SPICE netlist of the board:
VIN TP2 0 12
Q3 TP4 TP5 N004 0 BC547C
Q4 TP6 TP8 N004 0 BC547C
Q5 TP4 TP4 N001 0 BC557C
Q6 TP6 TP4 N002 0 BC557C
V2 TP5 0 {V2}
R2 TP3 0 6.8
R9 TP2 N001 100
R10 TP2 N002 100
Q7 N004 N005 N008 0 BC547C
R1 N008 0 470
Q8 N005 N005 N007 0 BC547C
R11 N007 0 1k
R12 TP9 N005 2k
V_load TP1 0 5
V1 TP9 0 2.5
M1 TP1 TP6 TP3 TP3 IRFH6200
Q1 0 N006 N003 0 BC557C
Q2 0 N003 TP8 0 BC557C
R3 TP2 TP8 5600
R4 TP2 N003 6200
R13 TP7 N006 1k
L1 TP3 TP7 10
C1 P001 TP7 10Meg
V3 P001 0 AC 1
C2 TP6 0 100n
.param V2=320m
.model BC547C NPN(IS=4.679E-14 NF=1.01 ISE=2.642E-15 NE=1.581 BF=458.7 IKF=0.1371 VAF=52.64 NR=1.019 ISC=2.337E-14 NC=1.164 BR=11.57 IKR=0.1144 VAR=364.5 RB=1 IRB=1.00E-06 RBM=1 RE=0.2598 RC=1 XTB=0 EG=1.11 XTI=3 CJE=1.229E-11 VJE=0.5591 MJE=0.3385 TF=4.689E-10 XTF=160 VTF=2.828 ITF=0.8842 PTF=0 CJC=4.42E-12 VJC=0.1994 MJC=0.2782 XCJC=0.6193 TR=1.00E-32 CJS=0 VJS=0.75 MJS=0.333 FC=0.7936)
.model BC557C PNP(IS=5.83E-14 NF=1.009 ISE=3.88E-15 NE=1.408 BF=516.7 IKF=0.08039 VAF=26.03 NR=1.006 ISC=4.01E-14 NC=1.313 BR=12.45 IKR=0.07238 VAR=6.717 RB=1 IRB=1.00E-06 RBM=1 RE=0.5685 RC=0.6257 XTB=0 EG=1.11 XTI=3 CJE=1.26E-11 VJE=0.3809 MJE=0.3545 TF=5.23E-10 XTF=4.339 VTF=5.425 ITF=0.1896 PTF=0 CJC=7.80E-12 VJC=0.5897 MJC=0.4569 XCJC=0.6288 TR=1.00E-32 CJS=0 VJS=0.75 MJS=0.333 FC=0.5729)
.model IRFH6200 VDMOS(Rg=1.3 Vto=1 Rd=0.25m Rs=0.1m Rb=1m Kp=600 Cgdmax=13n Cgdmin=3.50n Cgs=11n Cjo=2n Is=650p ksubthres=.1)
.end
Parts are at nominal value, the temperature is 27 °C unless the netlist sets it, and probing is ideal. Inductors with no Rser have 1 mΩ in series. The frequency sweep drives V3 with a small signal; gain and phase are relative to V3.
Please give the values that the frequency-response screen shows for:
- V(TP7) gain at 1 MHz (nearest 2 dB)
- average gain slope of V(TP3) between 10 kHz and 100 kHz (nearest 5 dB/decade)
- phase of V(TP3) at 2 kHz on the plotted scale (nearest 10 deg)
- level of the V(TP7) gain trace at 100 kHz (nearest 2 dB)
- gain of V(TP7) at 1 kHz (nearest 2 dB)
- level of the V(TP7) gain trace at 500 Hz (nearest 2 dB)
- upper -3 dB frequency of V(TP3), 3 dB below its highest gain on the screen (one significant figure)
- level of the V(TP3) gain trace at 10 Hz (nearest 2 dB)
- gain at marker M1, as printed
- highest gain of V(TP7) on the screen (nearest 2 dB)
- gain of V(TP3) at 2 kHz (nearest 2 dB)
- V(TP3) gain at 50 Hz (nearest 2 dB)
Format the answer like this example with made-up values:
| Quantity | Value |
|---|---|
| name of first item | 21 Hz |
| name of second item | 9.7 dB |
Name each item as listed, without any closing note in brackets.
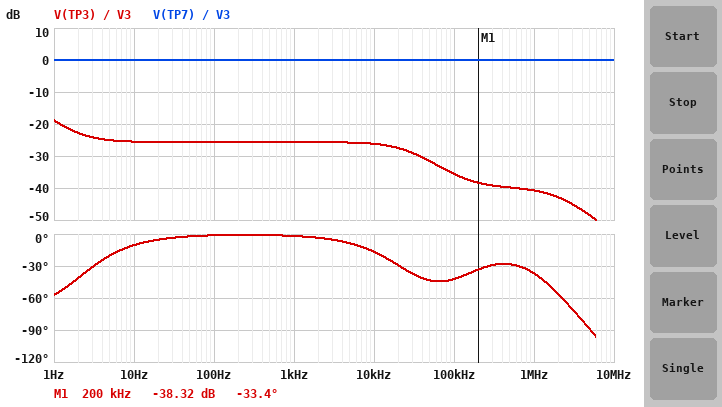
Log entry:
| Quantity | Value |
|---|---|
| V(TP7) gain at 1 MHz | 0 dB |
| average gain slope of V(TP3) between 10 kHz and 100 kHz | -10 dB/decade |
| phase of V(TP3) at 2 kHz on the plotted scale | 0 deg |
| level of the V(TP7) gain trace at 100 kHz | 0 dB |
| gain of V(TP7) at 1 kHz | 0 dB |
| level of the V(TP7) gain trace at 500 Hz | 0 dB |
| upper -3 dB frequency of V(TP3), 3 dB below its highest gain on the screen | 2 Hz |
| level of the V(TP3) gain trace at 10 Hz | -26 dB |
| gain at marker M1, as printed | -38.32 dB |
| highest gain of V(TP7) on the screen | 0 dB |
| gain of V(TP3) at 2 kHz | -26 dB |
| V(TP3) gain at 50 Hz | -26 dB |
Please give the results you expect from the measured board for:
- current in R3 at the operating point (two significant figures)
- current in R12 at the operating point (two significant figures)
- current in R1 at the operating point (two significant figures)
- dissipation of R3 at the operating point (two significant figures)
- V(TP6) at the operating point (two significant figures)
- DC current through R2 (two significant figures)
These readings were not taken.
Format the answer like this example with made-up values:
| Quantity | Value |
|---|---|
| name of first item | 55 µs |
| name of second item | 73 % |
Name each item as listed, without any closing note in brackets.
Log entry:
| Quantity | Value |
|---|---|
| current in R3 at the operating point | 1.9 mA |
| current in R12 at the operating point | 660 µA |
| current in R1 at the operating point | 1.2 mA |
| dissipation of R3 at the operating point | 21 mW |
| V(TP6) at the operating point | 570 mV |
| DC current through R2 | 480 µA |
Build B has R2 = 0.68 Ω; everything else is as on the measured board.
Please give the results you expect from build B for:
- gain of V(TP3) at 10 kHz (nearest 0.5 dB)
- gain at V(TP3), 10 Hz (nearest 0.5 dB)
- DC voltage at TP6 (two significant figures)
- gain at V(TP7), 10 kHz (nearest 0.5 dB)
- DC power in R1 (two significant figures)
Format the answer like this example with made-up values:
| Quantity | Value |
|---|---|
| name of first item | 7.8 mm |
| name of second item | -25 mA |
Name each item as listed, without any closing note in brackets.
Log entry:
| Quantity | Value |
|---|---|
| gain of V(TP3) at 10 kHz | -45.5 dB |
| gain at V(TP3), 10 Hz | -45.0 dB |
| DC voltage at TP6 | 560 mV |
| gain at V(TP7), 10 kHz | 0 dB |
| DC power in R1 | 630 µW |
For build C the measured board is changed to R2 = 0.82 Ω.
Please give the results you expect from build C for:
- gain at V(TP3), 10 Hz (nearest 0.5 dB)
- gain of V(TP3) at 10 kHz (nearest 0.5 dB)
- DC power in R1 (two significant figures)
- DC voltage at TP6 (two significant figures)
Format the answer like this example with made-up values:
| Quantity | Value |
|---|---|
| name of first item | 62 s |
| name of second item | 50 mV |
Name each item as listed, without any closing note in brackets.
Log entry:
| Quantity | Value |
|---|---|
| gain at V(TP3), 10 Hz | -43.5 dB |
| gain of V(TP3) at 10 kHz | -44.0 dB |
| DC power in R1 | 630 µW |
| DC voltage at TP6 | 560 mV |
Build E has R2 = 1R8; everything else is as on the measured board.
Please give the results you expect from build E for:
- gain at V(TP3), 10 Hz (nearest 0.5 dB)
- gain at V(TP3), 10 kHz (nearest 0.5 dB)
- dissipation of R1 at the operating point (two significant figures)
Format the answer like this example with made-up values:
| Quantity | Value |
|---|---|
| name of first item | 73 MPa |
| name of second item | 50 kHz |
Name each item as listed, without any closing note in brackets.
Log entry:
| Quantity | Value |
|---|---|
| gain at V(TP3), 10 Hz | -36.5 dB |
| gain at V(TP3), 10 kHz | -37.5 dB |
| dissipation of R1 at the operating point | 630 µW |
